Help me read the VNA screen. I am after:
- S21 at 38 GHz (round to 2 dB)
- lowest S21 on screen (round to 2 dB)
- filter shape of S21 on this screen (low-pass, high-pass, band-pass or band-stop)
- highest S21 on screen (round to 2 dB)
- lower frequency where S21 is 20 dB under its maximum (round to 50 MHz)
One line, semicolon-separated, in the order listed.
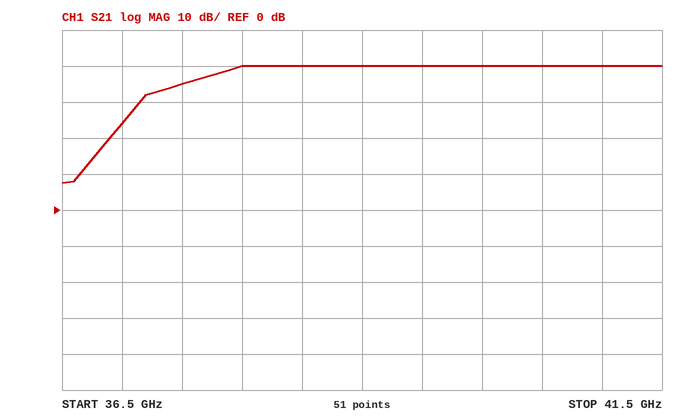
40 dB; 8 dB; high-pass; 40 dB; 36.90 GHz
